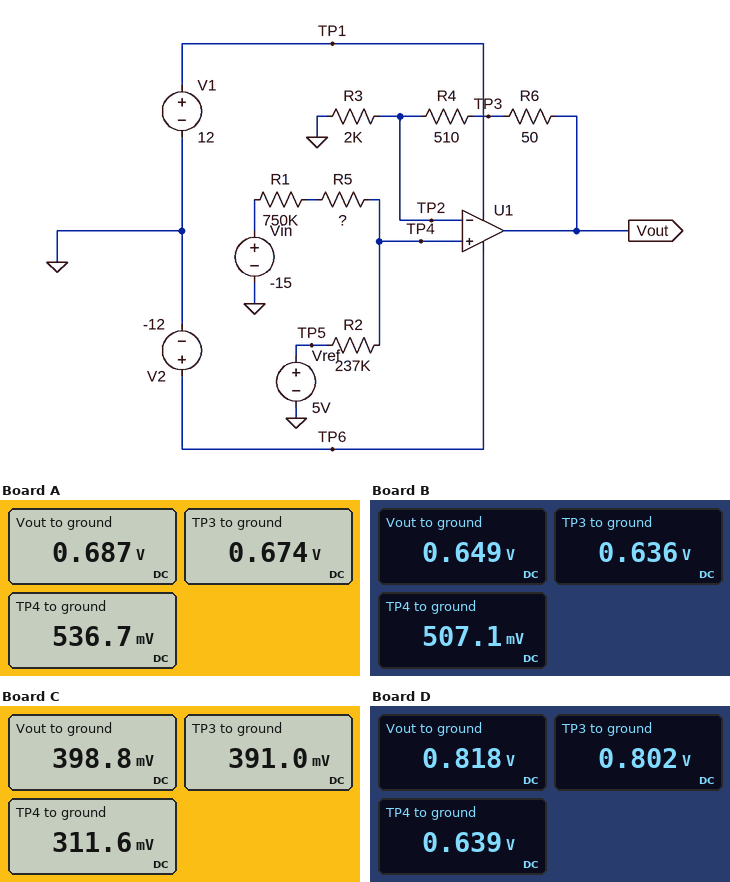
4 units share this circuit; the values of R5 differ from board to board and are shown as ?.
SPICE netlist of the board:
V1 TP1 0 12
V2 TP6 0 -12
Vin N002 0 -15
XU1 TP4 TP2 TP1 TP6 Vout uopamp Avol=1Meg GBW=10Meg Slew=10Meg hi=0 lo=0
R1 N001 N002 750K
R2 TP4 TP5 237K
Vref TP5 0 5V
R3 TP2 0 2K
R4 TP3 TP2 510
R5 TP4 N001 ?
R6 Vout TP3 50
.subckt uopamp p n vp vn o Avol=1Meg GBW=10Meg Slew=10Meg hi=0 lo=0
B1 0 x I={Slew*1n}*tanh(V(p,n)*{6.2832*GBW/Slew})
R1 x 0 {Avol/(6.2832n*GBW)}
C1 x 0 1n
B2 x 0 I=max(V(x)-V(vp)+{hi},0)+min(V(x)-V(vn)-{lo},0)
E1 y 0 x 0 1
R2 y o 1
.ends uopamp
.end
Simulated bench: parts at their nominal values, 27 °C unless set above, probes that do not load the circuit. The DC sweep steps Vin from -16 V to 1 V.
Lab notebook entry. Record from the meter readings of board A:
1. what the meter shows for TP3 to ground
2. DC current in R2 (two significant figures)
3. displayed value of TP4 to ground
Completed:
0.674 V
19 µA
536.7 mV
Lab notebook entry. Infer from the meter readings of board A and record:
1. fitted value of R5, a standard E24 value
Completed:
75 kΩ
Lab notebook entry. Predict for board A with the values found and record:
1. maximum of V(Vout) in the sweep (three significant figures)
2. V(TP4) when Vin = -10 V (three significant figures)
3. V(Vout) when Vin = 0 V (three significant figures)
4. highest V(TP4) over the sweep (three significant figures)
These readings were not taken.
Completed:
5.26 V
1.65 V
4.97 V
4.11 V
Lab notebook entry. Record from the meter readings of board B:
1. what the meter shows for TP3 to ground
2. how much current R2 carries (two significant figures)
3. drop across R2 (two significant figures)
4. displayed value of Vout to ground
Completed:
0.636 V
19 µA
4.5 V
0.649 V
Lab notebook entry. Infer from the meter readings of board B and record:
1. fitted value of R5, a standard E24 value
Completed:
68 kΩ
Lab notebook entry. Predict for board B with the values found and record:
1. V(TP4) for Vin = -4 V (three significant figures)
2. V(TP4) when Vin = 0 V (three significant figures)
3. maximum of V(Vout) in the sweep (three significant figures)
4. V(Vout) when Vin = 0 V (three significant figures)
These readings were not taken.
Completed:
2.98 V
3.88 V
5.25 V
4.96 V
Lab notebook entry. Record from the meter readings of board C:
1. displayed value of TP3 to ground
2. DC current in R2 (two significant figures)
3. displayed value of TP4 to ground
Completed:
391.0 mV
20 µA
311.6 mV
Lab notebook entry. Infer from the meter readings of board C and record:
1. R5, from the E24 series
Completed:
24 kΩ
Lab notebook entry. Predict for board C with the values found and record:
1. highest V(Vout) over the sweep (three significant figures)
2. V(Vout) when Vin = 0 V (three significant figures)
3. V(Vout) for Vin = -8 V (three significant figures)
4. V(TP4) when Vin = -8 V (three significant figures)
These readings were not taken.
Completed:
5.20 V
4.90 V
2.50 V
1.95 V
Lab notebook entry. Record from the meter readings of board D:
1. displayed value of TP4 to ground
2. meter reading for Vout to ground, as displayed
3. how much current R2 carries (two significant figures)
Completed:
0.639 V
0.818 V
18 µA
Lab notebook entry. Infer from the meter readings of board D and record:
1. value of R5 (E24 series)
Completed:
100 kΩ
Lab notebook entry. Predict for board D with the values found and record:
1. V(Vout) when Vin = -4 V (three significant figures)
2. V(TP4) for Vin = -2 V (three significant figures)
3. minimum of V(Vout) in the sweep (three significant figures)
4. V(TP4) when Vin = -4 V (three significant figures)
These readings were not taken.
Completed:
3.89 V
3.47 V
539 mV
3.04 V
